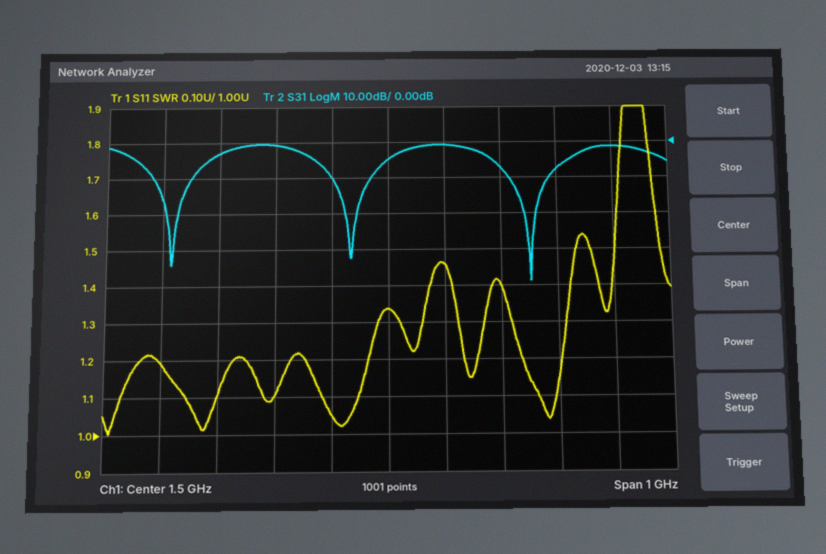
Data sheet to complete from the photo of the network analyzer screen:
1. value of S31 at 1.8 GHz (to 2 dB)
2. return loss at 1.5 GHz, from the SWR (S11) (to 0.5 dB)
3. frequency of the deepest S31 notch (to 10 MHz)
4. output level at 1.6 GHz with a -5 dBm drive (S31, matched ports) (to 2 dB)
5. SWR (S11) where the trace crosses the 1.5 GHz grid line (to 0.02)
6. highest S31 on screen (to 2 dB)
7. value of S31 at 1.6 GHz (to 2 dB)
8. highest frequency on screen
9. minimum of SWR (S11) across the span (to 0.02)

-8 dB
17.0 dB
1.75 GHz
-6 dBm
1.34
0 dB
0 dB
2 GHz
1.00
